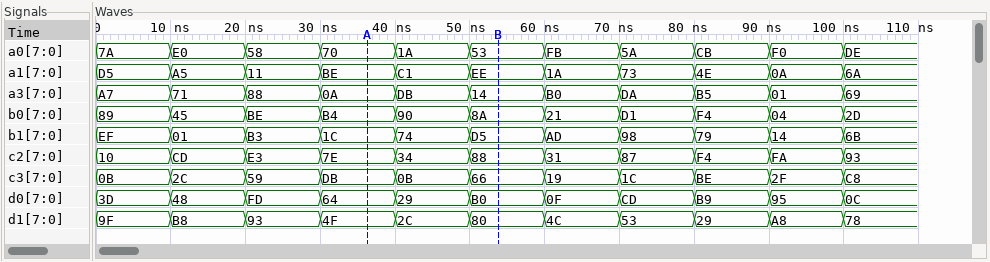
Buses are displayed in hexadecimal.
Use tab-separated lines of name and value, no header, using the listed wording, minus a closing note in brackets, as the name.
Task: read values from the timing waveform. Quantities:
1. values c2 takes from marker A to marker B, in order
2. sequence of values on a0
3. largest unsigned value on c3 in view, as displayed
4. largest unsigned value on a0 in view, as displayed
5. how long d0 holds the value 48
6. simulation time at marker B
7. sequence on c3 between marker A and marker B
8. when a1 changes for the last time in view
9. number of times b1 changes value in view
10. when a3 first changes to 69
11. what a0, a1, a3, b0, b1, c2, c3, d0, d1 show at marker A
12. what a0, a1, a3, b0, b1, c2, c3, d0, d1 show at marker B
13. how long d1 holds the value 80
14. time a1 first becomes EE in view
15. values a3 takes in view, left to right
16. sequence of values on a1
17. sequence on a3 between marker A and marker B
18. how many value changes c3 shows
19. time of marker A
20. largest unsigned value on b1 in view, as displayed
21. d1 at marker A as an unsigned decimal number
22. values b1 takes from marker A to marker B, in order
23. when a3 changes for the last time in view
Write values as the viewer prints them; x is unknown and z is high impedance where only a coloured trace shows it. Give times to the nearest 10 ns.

values c2 takes from marker A to marker B, in order	7E, 34, 88
sequence of values on a0	7A, E0, 58, 70, 1A, 53, FB, 5A, CB, F0, DE
largest unsigned value on c3 in view, as displayed	DB
largest unsigned value on a0 in view, as displayed	FB
how long d0 holds the value 48	10 ns
simulation time at marker B	50 ns
sequence on c3 between marker A and marker B	DB, 0B, 66
when a1 changes for the last time in view	100 ns
number of times b1 changes value in view	10
when a3 first changes to 69	100 ns
what a0, a1, a3, b0, b1, c2, c3, d0, d1 show at marker A	a0=70, a1=BE, a3=0A, b0=B4, b1=1C, c2=7E, c3=DB, d0=64, d1=4F
what a0, a1, a3, b0, b1, c2, c3, d0, d1 show at marker B	a0=53, a1=EE, a3=14, b0=8A, b1=D5, c2=88, c3=66, d0=B0, d1=80
how long d1 holds the value 80	10 ns
time a1 first becomes EE in view	50 ns
values a3 takes in view, left to right	A7, 71, 88, 0A, DB, 14, B0, DA, B5, 01, 69
sequence of values on a1	D5, A5, 11, BE, C1, EE, 1A, 73, 4E, 0A, 6A
sequence on a3 between marker A and marker B	0A, DB, 14
how many value changes c3 shows	10
time of marker A	40 ns
largest unsigned value on b1 in view, as displayed	EF
d1 at marker A as an unsigned decimal number	79
values b1 takes from marker A to marker B, in order	1C, 74, D5
when a3 changes for the last time in view	100 ns
